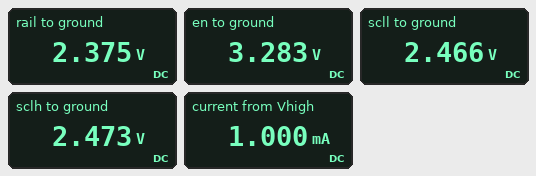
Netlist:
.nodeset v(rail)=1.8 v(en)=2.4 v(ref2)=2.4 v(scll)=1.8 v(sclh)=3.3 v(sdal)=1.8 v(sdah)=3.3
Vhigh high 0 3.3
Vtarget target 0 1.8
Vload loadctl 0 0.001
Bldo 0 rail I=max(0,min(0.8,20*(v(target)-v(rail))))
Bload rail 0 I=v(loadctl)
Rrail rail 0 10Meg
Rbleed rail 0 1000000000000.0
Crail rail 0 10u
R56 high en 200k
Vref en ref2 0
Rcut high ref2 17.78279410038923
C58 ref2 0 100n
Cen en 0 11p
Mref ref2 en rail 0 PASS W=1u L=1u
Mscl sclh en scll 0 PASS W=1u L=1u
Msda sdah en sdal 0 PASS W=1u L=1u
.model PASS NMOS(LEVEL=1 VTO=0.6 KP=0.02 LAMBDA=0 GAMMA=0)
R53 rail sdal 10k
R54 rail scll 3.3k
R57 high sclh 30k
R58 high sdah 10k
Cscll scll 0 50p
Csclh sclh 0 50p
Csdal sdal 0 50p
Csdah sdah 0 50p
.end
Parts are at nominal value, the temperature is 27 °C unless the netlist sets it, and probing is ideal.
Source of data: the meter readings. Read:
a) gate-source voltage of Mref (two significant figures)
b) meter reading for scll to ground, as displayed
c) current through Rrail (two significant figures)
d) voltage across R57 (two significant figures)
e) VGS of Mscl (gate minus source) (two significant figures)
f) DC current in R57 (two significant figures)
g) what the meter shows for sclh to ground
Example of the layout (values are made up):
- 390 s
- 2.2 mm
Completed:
- 910 mV
- 2.466 V
- 240 nA
- 830 mV
- 820 mV
- 28 µA
- 2.473 V
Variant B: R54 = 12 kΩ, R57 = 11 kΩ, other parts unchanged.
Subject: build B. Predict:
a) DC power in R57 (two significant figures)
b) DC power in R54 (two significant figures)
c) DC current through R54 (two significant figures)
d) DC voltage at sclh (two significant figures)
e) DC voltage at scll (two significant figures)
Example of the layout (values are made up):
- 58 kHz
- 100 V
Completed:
- 5.2 µW
- 5.7 µW
- 22 µA
- 3.1 V
- 2.6 V
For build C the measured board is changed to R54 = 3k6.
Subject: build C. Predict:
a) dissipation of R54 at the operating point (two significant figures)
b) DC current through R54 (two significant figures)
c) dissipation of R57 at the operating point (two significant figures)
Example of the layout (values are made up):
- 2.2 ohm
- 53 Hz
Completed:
- 2.7 µW
- 27 µA
- 22 µW
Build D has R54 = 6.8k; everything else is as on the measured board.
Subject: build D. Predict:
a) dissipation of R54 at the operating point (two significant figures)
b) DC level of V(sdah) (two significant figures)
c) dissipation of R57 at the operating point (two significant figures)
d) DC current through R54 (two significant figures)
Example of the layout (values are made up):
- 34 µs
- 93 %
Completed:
- 4.2 µW
- 3.0 V
- 19 µW
- 25 µA
